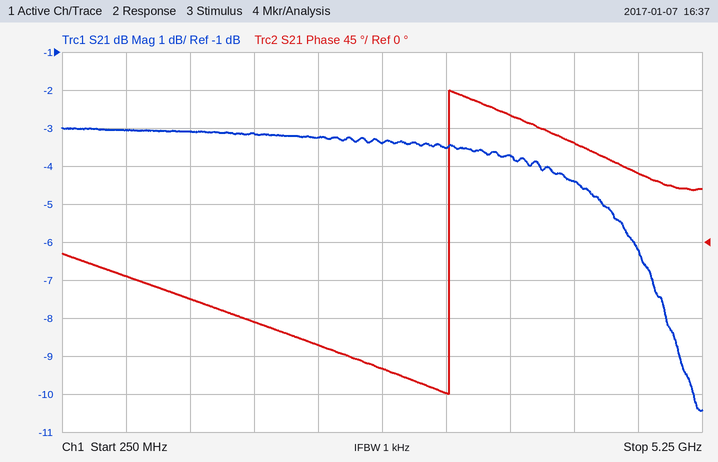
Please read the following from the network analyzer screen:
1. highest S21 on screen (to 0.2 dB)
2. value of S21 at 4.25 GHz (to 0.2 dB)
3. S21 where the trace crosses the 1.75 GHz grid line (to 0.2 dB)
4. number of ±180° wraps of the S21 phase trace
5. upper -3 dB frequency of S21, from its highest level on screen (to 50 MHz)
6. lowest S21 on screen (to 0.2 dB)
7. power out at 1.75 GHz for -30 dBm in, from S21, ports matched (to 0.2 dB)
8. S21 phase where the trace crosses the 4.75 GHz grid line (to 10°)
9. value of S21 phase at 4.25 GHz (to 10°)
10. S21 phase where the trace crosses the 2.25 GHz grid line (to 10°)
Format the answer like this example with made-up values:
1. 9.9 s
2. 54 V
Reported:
1. -3.0 dB
2. -4.4 dB
3. -3.2 dB
4. 1
5. 4.70 GHz
6. -10.4 dB
7. -33.2 dBm
8. 80°
9. 120°
10. -120°
